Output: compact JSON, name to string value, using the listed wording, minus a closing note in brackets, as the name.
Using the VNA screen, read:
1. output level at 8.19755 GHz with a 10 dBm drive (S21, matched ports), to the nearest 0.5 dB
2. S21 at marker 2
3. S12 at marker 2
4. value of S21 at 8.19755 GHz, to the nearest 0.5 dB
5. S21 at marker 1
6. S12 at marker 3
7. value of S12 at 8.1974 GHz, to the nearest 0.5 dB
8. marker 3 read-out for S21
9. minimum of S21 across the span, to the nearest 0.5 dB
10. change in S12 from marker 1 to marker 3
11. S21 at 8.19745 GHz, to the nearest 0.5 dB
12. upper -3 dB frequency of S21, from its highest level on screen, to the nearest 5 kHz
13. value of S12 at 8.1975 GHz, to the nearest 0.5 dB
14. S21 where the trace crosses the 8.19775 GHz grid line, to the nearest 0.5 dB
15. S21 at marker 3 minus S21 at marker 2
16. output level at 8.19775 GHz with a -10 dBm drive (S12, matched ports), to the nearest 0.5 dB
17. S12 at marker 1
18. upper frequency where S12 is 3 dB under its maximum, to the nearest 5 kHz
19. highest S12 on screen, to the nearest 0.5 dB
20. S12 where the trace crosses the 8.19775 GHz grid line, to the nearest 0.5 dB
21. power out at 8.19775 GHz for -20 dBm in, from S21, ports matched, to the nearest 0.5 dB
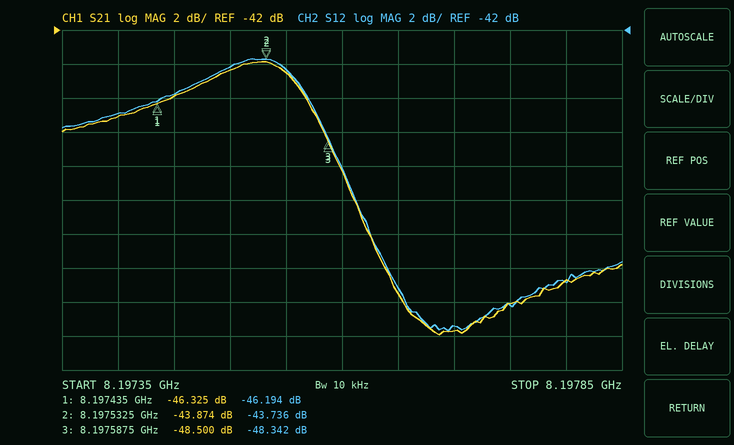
{"output level at 8.19755 GHz with a 10 dBm drive (S21, matched ports), to the nearest 0.5 dB": "-34.5 dBm", "S21 at marker 2": "-43.874 dB", "S12 at marker 2": "-43.736 dB", "value of S21 at 8.19755 GHz, to the nearest 0.5 dB": "-44.5 dB", "S21 at marker 1": "-46.325 dB", "S12 at marker 3": "-48.342 dB", "value of S12 at 8.1974 GHz, to the nearest 0.5 dB": "-47.0 dB", "marker 3 read-out for S21": "-48.500 dB", "minimum of S21 across the span, to the nearest 0.5 dB": "-60.0 dB", "change in S12 from marker 1 to marker 3": "-2.148 dB", "S21 at 8.19745 GHz, to the nearest 0.5 dB": "-46.0 dB", "upper -3 dB frequency of S21, from its highest level on screen, to the nearest 5 kHz": "8.197575 GHz", "value of S12 at 8.1975 GHz, to the nearest 0.5 dB": "-44.0 dB", "S21 where the trace crosses the 8.19775 GHz grid line, to the nearest 0.5 dB": "-58.0 dB", "S21 at marker 3 minus S21 at marker 2": "-4.626 dB", "output level at 8.19775 GHz with a -10 dBm drive (S12, matched ports), to the nearest 0.5 dB": "-68.0 dBm", "S12 at marker 1": "-46.194 dB", "upper frequency where S12 is 3 dB under its maximum, to the nearest 5 kHz": "8.197575 GHz", "highest S12 on screen, to the nearest 0.5 dB": "-43.5 dB", "S12 where the trace crosses the 8.19775 GHz grid line, to the nearest 0.5 dB": "-58.0 dB", "power out at 8.19775 GHz for -20 dBm in, from S21, ports matched, to the nearest 0.5 dB": "-78.0 dBm"}
